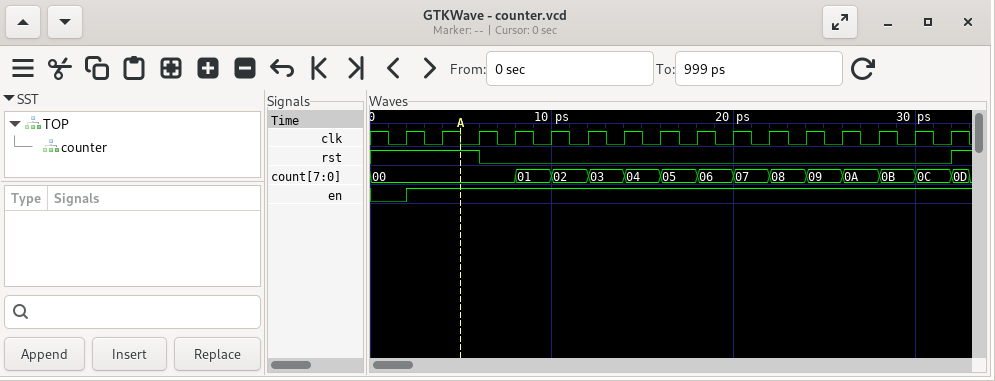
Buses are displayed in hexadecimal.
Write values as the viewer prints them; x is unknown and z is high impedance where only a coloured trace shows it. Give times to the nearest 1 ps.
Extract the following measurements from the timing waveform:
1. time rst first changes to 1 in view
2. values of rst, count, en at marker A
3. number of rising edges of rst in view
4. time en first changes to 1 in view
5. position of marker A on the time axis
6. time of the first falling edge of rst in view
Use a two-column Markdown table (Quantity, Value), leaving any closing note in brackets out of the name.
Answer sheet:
| Quantity | Value |
|---|---|
| time rst first changes to 1 in view | 32 ps |
| values of rst, count, en at marker A | rst=1, count=00, en=1 |
| number of rising edges of rst in view | 1 |
| time en first changes to 1 in view | 2 ps |
| position of marker A on the time axis | 5 ps |
| time of the first falling edge of rst in view | 6 ps |
